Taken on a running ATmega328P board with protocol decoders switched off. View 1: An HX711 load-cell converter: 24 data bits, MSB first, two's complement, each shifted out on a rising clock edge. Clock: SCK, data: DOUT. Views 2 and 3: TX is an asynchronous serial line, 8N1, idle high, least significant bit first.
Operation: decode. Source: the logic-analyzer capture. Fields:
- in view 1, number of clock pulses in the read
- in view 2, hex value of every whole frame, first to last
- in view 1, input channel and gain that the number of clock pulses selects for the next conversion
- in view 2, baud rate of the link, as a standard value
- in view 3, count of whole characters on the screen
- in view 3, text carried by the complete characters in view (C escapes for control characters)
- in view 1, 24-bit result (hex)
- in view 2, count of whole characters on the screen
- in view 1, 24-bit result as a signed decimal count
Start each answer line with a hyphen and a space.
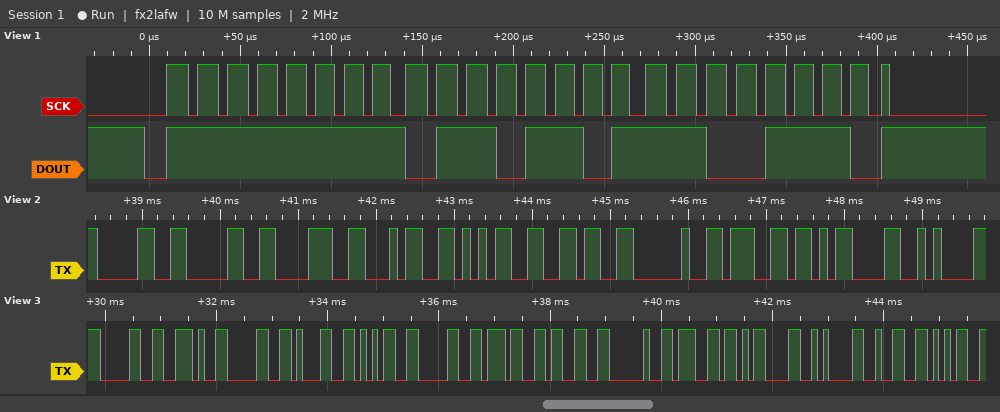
- 25
- 30 30 38 34 35 36 20 67 0D 0A
- channel A, gain 128
- 9600 baud
- 14
- "0.015073 g\r\n25"
- 0xFF6DCE
- 10
- -37426
